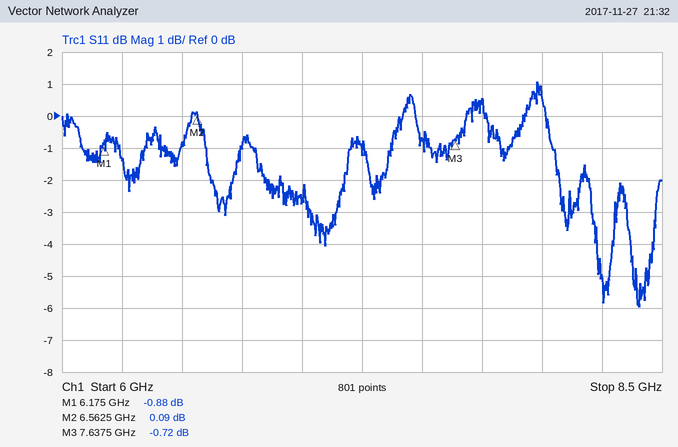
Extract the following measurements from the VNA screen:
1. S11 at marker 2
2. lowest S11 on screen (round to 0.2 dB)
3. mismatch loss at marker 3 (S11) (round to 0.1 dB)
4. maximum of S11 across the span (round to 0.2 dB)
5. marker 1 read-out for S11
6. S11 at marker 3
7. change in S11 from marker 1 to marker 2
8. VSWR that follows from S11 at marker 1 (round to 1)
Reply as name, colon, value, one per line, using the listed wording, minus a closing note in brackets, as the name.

S11 at marker 2: 0.09 dB
lowest S11 on screen: -6.0 dB
mismatch loss at marker 3 (S11): 8.2 dB
maximum of S11 across the span: 1.0 dB
marker 1 read-out for S11: -0.88 dB
S11 at marker 3: -0.72 dB
change in S11 from marker 1 to marker 2: 0.97 dB
VSWR that follows from S11 at marker 1: 20
